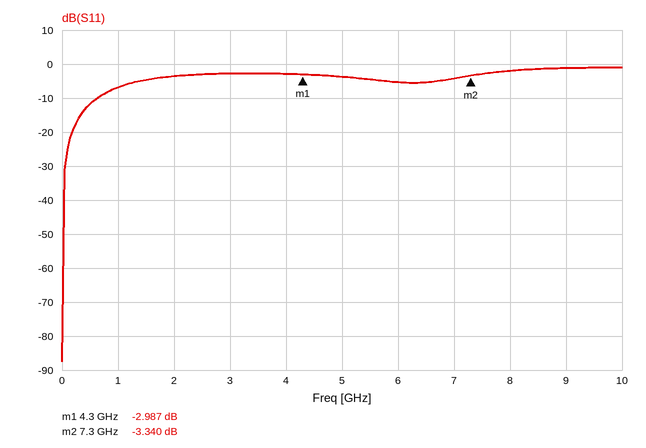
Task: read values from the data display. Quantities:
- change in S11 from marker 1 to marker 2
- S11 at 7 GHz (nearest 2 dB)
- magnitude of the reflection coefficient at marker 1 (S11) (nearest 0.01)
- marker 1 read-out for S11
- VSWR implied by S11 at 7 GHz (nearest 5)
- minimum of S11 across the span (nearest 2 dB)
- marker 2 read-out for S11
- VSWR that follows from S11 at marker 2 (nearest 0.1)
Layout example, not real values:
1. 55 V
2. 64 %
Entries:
1. -0.353 dB
2. -4 dB
3. 0.71
4. -2.987 dB
5. 5
6. -88 dB
7. -3.340 dB
8. 5.3
